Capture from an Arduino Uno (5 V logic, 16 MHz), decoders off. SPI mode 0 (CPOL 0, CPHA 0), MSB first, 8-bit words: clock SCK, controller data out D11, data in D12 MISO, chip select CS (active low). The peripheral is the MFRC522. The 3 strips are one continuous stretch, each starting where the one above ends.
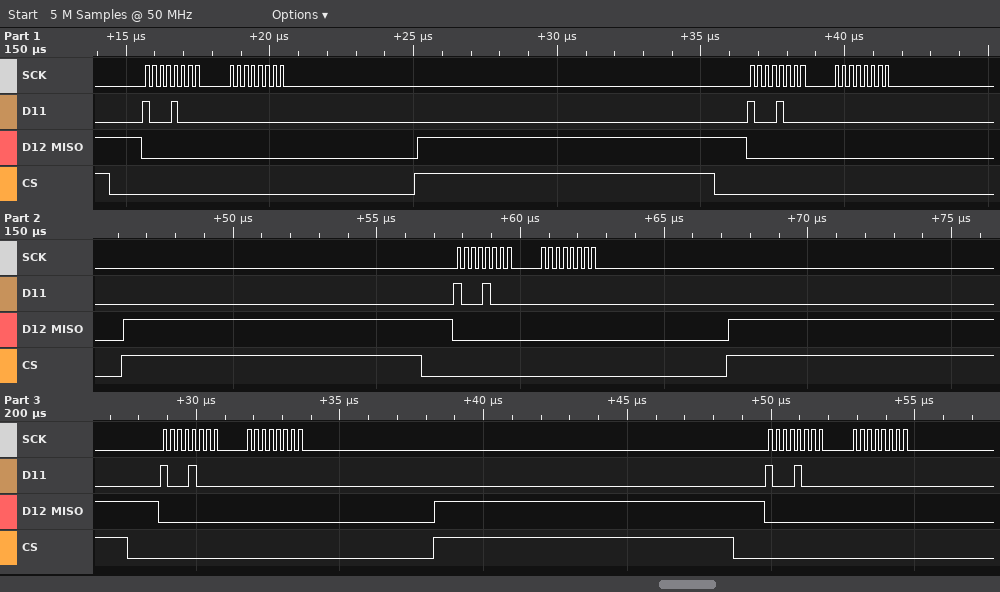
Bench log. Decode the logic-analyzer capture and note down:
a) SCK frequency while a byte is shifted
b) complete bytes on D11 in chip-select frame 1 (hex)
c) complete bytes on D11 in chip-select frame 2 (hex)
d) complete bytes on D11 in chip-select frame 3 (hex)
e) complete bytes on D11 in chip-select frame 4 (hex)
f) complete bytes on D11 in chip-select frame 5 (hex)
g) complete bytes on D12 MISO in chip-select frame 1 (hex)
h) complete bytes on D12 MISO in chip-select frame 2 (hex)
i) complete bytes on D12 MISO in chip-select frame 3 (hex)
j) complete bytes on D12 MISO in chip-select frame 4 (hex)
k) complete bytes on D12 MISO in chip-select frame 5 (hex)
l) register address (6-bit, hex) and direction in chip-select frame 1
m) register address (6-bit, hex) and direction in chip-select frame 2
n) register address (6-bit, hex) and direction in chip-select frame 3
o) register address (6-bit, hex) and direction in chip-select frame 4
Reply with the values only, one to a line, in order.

4 MHz
0x88 0x00
0x88 0x00
0x88 0x00
0x88 0x00
0x88 0x00
0x00 0x00
0x00 0x00
0x00 0x00
0x00 0x00
0x00 0x00
0x04 read
0x04 read
0x04 read
0x04 read
